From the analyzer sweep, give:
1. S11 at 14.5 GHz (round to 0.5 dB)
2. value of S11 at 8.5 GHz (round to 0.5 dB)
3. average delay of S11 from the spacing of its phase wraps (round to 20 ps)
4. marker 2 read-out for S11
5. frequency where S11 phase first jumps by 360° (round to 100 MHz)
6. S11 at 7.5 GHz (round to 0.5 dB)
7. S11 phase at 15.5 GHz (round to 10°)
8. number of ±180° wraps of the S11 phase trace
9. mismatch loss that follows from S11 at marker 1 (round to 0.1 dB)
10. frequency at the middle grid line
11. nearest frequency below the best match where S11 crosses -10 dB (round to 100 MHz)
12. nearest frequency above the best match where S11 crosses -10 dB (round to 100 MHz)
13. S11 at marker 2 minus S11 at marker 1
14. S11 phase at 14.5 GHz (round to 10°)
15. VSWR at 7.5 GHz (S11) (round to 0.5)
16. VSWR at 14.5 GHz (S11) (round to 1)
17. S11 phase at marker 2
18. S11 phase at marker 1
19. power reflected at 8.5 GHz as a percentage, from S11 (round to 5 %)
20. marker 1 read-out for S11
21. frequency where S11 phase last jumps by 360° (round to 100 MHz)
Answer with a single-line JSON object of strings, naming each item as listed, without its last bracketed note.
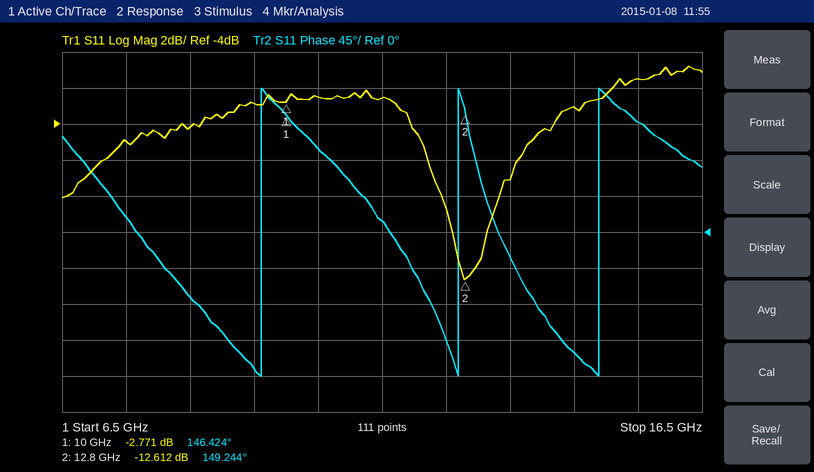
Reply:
{"S11 at 14.5 GHz": "-3.0 dB", "value of S11 at 8.5 GHz": "-4.0 dB", "average delay of S11 from the spacing of its phase wraps": "380 ps", "marker 2 read-out for S11": "-12.612 dB", "frequency where S11 phase first jumps by 360°": "9.6 GHz", "S11 at 7.5 GHz": "-5.0 dB", "S11 phase at 15.5 GHz": "140°", "number of ±180° wraps of the S11 phase trace": "3", "mismatch loss that follows from S11 at marker 1": "3.3 dB", "frequency at the middle grid line": "11.5 GHz", "nearest frequency below the best match where S11 crosses -10 dB": "12.6 GHz", "nearest frequency above the best match where S11 crosses -10 dB": "13.1 GHz", "S11 at marker 2 minus S11 at marker 1": "-9.841 dB", "S11 phase at 14.5 GHz": "-150°", "VSWR at 7.5 GHz (S11)": "3.5", "VSWR at 14.5 GHz (S11)": "6", "S11 phase at marker 2": "149.244°", "S11 phase at marker 1": "146.424°", "power reflected at 8.5 GHz as a percentage, from S11": "40 %", "marker 1 read-out for S11": "-2.771 dB", "frequency where S11 phase last jumps by 360°": "14.9 GHz"}
